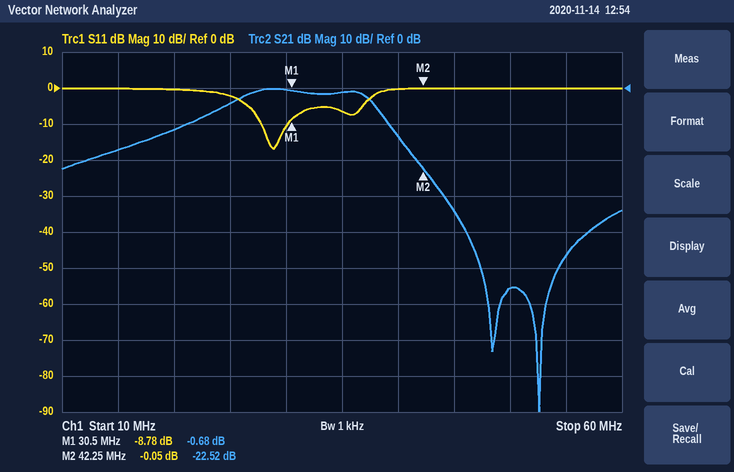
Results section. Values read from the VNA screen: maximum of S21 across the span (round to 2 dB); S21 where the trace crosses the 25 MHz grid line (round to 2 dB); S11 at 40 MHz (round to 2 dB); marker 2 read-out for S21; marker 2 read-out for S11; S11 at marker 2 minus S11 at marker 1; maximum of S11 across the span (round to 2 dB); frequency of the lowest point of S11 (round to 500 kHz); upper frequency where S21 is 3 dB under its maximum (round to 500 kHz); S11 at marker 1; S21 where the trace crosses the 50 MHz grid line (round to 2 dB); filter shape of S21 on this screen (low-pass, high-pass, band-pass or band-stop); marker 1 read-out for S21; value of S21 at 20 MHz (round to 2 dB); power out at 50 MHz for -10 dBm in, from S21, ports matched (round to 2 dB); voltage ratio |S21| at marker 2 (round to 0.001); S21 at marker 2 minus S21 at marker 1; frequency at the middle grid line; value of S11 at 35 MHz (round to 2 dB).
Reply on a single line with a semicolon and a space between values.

0 dB; -4 dB; 0 dB; -22.52 dB; -0.05 dB; 8.73 dB; 0 dB; 29.0 MHz; 37.5 MHz; -8.78 dB; -56 dB; band-pass; -0.68 dB; -12 dB; -66 dBm; 0.075; -21.84 dB; 35 MHz; -6 dB
